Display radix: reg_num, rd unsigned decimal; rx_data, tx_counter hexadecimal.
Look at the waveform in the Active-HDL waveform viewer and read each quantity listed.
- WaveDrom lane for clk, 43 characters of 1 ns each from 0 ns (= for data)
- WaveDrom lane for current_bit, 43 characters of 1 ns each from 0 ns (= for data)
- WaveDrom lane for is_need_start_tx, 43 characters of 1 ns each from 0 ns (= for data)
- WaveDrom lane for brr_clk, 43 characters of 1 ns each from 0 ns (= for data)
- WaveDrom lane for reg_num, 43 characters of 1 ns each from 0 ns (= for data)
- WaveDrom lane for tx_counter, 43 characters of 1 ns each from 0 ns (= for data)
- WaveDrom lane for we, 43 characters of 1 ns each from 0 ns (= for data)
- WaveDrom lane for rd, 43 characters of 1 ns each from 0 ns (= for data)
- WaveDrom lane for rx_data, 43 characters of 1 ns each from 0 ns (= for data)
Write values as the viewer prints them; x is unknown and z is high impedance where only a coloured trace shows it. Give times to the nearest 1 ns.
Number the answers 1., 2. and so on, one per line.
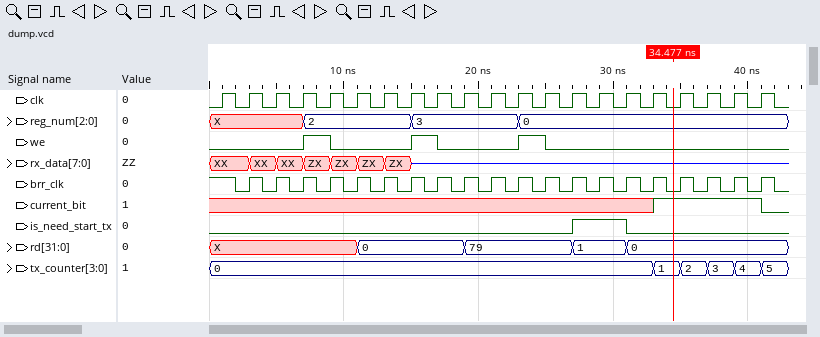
1. {name: 'clk', wave: '0101010101010101010101010101010101010101010'}
2. {name: 'current_bit', wave: 'x................................1.......0.'}
3. {name: 'is_need_start_tx', wave: '0..........................1...0...........'}
4. {name: 'brr_clk', wave: '1.01010101010101010101010101010101010101010'}
5. {name: 'reg_num', wave: 'x......=.......=.......=...................', data: '2 3 0'}
6. {name: 'tx_counter', wave: '=................................=.=.=.=.=.', data: '0 1 2 3 4 5'}
7. {name: 'we', wave: '0......1.0.....1.0.....1.0.................'}
8. {name: 'rd', wave: 'x..........=.......=.......=...=...........', data: '0 79 1 0'}
9. {name: 'rx_data', wave: '=..=.=.=.=.=.=.z...........................', data: 'XX XX XX ZX ZX ZX ZX'}
